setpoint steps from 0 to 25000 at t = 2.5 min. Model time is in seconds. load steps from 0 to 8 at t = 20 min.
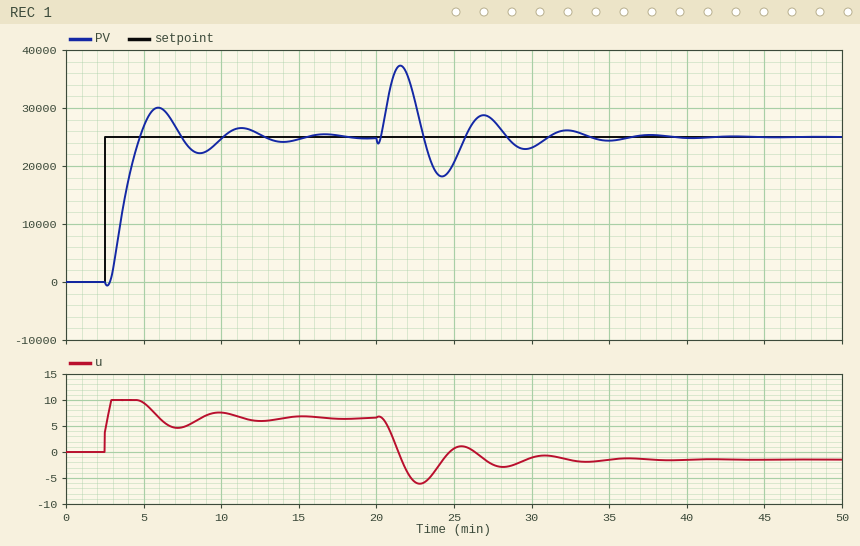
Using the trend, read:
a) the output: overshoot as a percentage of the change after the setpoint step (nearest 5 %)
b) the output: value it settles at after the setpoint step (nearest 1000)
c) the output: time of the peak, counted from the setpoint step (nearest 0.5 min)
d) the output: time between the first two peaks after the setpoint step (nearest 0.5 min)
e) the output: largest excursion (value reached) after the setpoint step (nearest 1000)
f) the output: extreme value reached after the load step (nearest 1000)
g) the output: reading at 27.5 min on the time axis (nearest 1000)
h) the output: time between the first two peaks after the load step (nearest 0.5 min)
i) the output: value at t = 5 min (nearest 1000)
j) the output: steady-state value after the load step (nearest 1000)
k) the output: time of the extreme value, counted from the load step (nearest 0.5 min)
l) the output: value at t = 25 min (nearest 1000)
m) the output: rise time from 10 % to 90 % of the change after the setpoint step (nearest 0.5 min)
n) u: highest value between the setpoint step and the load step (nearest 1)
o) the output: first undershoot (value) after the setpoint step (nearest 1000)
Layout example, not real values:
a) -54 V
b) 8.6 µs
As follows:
a) 20 %
b) 25000
c) 3.5 min
d) 5.5 min
e) 30000
f) 37000
g) 28000
h) 5.5 min
i) 27000
j) 25000
k) 1.5 min
l) 21000
m) 1.5 min
n) 10
o) 22000
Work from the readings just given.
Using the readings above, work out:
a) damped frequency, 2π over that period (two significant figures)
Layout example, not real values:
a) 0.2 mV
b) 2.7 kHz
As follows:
a) 1.1 rad/min
